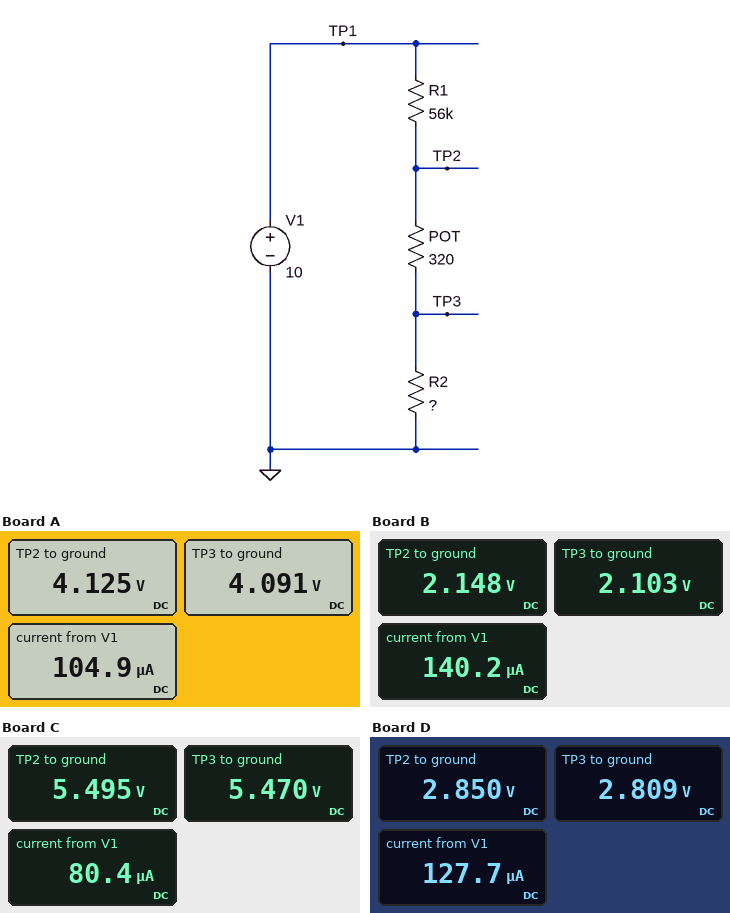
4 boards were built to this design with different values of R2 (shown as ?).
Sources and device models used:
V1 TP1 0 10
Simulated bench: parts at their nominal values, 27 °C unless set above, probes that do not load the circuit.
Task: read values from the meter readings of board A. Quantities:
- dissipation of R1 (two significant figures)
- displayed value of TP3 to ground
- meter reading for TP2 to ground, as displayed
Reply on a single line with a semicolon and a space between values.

620 µW; 4.091 V; 4.125 V
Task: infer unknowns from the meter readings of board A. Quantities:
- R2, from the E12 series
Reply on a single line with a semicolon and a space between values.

39 kΩ
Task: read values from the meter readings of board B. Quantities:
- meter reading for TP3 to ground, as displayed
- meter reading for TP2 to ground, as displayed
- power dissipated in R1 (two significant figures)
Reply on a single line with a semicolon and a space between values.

2.103 V; 2.148 V; 1.1 mW
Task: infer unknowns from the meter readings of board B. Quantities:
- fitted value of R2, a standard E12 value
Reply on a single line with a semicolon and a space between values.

15 kΩ
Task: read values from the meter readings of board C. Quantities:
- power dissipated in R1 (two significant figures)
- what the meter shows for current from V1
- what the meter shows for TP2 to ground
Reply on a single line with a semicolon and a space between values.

360 µW; 80.4 µA; 5.495 V
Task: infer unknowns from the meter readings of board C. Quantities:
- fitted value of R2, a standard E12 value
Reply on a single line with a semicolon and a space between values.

68 kΩ
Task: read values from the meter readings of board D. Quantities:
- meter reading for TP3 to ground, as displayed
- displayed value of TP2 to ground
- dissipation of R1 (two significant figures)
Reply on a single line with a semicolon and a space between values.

2.809 V; 2.850 V; 910 µW
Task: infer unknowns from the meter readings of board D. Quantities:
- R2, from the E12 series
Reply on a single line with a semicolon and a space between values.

22 kΩ
